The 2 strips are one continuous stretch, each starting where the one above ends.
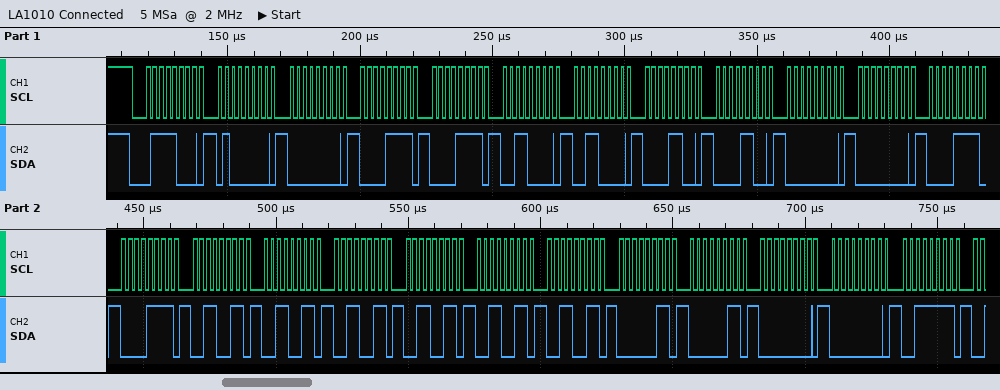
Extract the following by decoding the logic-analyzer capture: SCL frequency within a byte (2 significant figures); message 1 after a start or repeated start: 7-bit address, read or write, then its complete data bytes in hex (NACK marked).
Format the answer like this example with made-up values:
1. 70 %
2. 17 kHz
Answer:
1. 400 kHz
2. 0x3C write: 40 00 0F 0F 30 30 0C 0C 00 00 0F 0F 33 33 33 33 33 33 03 03 00 00 3F
